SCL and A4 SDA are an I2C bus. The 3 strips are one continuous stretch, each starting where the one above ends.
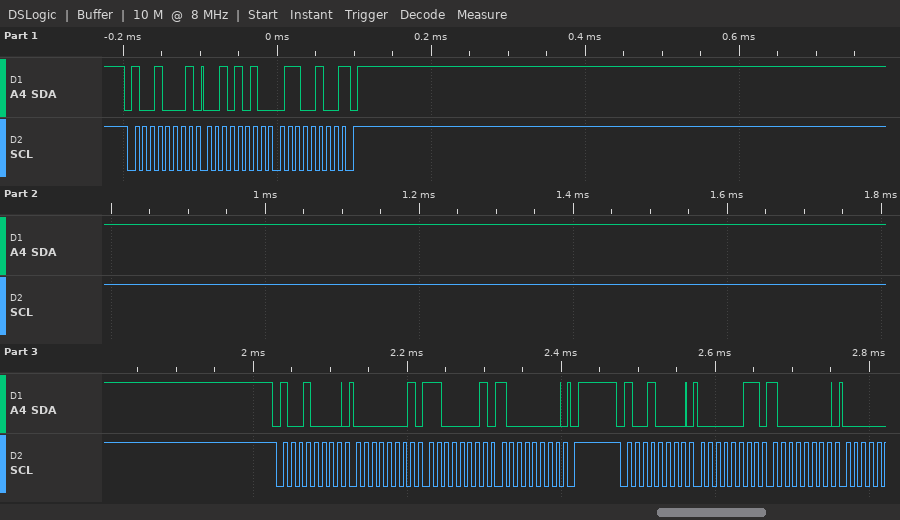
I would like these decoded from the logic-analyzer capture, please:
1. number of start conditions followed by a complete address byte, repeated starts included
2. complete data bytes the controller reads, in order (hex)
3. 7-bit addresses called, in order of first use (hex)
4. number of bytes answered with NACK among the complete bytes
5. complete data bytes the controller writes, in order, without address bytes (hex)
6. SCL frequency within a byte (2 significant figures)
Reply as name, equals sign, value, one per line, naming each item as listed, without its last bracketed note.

number of start conditions followed by a complete address byte, repeated starts included = 3
complete data bytes the controller reads, in order = 2A 64
7-bit addresses called, in order of first use = 0x48
number of bytes answered with NACK among the complete bytes = 1
complete data bytes the controller writes, in order, without address bytes = 01 C1 80 03 80
SCL frequency within a byte = 100 kHz
